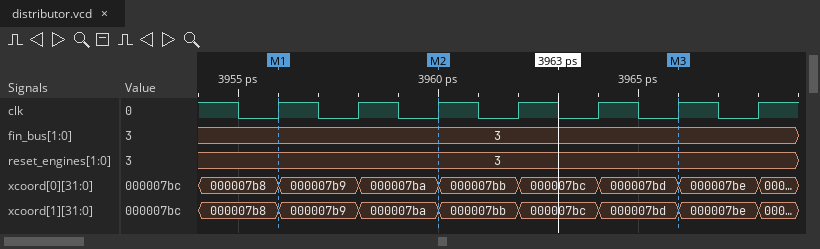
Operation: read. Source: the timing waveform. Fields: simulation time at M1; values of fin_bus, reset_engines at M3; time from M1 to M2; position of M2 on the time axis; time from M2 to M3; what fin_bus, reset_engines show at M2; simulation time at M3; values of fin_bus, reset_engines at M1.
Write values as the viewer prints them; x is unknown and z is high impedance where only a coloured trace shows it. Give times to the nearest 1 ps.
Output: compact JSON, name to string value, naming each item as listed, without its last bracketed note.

{"simulation time at M1": "3956 ps", "values of fin_bus, reset_engines at M3": "fin_bus=3, reset_engines=3", "time from M1 to M2": "4 ps", "position of M2 on the time axis": "3960 ps", "time from M2 to M3": "6 ps", "what fin_bus, reset_engines show at M2": "fin_bus=3, reset_engines=3", "simulation time at M3": "3966 ps", "values of fin_bus, reset_engines at M1": "fin_bus=3, reset_engines=3"}
